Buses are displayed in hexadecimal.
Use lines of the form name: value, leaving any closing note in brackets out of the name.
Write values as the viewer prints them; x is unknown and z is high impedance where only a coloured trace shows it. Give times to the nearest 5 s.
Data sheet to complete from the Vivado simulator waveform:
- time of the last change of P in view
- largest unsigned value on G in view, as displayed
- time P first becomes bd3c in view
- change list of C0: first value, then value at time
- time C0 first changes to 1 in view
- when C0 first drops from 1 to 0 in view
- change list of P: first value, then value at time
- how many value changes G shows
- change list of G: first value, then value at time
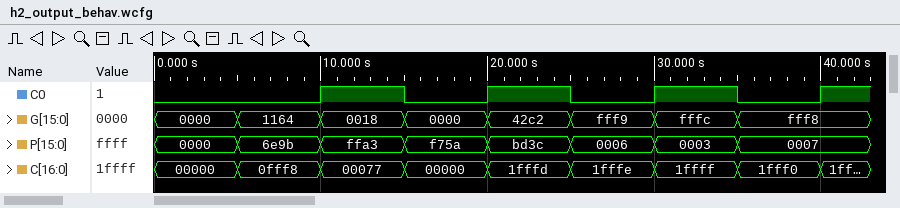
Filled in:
time of the last change of P in view: 35 s
largest unsigned value on G in view, as displayed: fffc
time P first becomes bd3c in view: 20 s
change list of C0: first value, then value at time: 0, 1 at 10 s, 0 at 15 s, 1 at 20 s, 0 at 25 s, 1 at 30 s, 0 at 35 s, 1 at 40 s
time C0 first changes to 1 in view: 10 s
when C0 first drops from 1 to 0 in view: 15 s
change list of P: first value, then value at time: 0000, 6e9b at 5 s, ffa3 at 10 s, f75a at 15 s, bd3c at 20 s, 0006 at 25 s, 0003 at 30 s, 0007 at 35 s
how many value changes G shows: 7
change list of G: first value, then value at time: 0000, 1164 at 5 s, 0018 at 10 s, 0000 at 15 s, 42c2 at 20 s, fff9 at 25 s, fffc at 30 s, fff8 at 35 s
